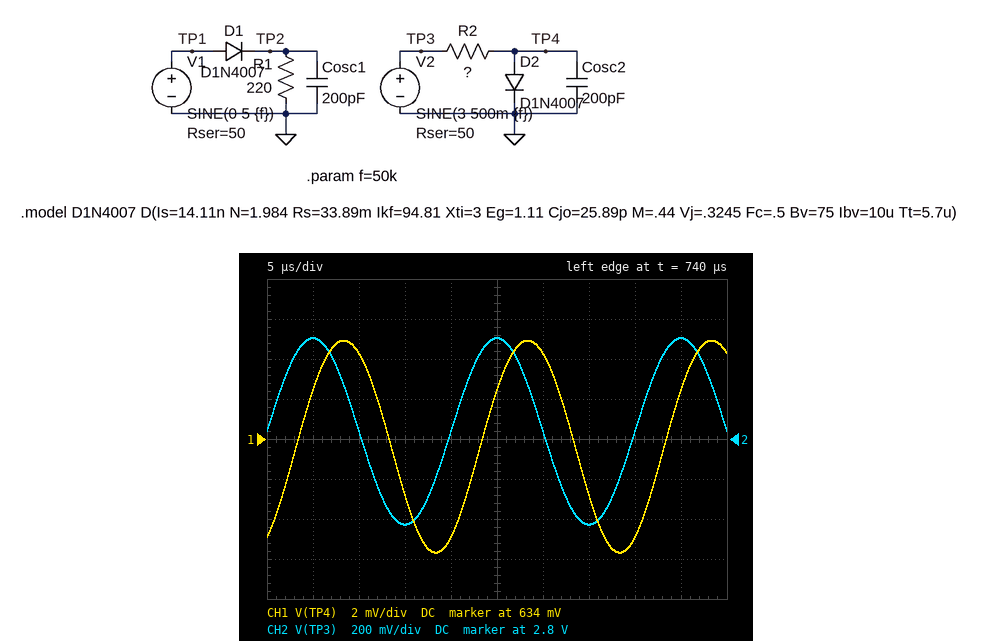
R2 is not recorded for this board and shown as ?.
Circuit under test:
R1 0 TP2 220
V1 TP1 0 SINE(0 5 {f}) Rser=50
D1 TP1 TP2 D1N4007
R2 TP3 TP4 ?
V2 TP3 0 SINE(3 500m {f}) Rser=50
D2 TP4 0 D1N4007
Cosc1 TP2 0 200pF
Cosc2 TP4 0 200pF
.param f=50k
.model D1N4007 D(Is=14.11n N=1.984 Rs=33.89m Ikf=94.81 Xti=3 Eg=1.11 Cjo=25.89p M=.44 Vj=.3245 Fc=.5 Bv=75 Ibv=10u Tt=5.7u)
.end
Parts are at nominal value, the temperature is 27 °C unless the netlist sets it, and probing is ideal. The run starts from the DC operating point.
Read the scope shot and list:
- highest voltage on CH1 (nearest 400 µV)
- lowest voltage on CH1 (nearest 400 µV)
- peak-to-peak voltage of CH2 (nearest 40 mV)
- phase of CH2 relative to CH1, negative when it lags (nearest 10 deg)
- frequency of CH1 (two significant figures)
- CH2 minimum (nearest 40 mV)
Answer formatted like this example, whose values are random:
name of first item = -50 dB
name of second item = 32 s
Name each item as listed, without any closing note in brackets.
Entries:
highest voltage on CH1 = 638.8 mV
lowest voltage on CH1 = 628.4 mV
peak-to-peak voltage of CH2 = 920 mV
phase of CH2 relative to CH1, negative when it lags = 60 deg
frequency of CH1 = 50 kHz
CH2 minimum = 2.36 V
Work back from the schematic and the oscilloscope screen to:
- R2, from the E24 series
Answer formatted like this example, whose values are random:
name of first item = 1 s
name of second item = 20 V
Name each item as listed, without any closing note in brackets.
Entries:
R2, from the E24 series = 680 Ω
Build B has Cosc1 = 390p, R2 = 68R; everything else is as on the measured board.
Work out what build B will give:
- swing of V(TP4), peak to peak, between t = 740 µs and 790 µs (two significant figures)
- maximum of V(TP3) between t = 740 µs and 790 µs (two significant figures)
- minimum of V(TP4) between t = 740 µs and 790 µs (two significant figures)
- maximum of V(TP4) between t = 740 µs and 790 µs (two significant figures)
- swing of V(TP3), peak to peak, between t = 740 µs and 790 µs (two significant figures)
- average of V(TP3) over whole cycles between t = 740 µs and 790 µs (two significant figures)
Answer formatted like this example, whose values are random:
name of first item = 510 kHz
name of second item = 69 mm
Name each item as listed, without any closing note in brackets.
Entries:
swing of V(TP4), peak to peak, between t = 740 µs and 790 µs = 11 mV
maximum of V(TP3) between t = 740 µs and 790 µs = 2.3 V
minimum of V(TP4) between t = 740 µs and 790 µs = 720 mV
maximum of V(TP4) between t = 740 µs and 790 µs = 730 mV
swing of V(TP3), peak to peak, between t = 740 µs and 790 µs = 580 mV
average of V(TP3) over whole cycles between t = 740 µs and 790 µs = 2.0 V
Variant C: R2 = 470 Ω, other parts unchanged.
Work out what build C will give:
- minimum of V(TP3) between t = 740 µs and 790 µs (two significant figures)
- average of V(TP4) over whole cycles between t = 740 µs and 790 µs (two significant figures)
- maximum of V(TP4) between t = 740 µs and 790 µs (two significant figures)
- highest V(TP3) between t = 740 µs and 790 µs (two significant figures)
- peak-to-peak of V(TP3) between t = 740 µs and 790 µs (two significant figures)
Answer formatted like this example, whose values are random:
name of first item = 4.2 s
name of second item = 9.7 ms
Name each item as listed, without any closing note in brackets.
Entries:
minimum of V(TP3) between t = 740 µs and 790 µs = 2.3 V
average of V(TP4) over whole cycles between t = 740 µs and 790 µs = 650 mV
maximum of V(TP4) between t = 740 µs and 790 µs = 660 mV
highest V(TP3) between t = 740 µs and 790 µs = 3.2 V
peak-to-peak of V(TP3) between t = 740 µs and 790 µs = 900 mV
